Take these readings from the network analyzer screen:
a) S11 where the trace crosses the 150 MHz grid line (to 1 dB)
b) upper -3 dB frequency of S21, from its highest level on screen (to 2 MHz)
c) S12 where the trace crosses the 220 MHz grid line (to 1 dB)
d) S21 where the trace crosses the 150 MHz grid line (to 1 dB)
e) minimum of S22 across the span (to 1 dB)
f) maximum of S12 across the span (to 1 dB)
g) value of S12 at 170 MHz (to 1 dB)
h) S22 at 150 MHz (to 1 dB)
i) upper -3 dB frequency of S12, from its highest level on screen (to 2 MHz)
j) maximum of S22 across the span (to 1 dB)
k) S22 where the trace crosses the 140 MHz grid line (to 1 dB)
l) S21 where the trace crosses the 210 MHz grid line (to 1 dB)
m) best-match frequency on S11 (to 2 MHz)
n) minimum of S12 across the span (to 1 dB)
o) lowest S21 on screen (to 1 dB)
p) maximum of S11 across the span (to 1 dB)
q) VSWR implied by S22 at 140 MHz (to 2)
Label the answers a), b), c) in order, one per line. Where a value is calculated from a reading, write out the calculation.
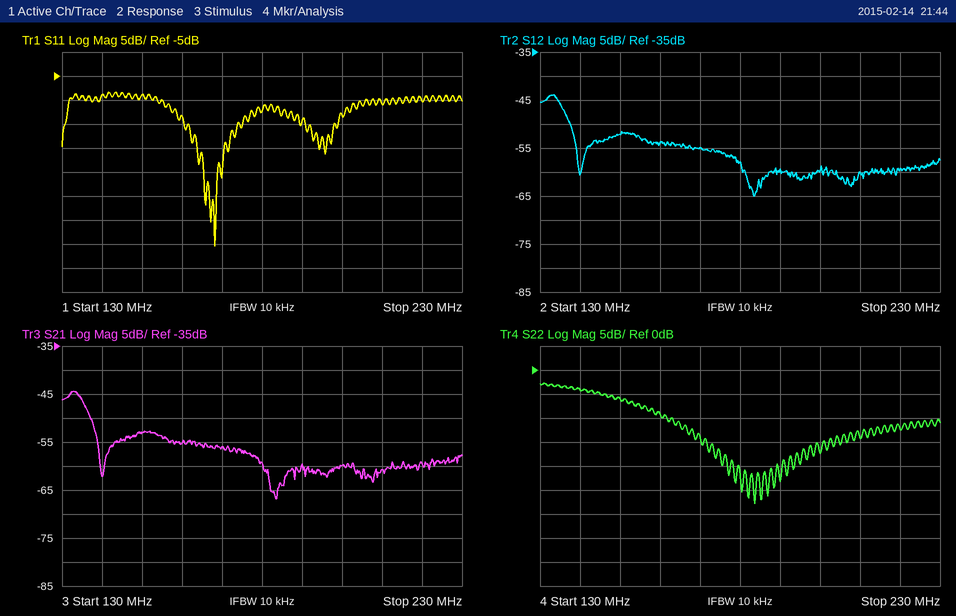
a) -9 dB
b) 136 MHz
c) -59 dB
d) -53 dB
e) -28 dB
f) -44 dB
g) -55 dB
h) -6 dB
i) 136 MHz
j) -3 dB
k) -4 dB
l) -61 dB
m) 168 MHz
n) -65 dB
o) -67 dB
p) -8 dB
q) |Γ| = 10^(-4/20) = 0.6310; VSWR = (1 + 0.6310)/(1 − 0.6310) ≈ 4
